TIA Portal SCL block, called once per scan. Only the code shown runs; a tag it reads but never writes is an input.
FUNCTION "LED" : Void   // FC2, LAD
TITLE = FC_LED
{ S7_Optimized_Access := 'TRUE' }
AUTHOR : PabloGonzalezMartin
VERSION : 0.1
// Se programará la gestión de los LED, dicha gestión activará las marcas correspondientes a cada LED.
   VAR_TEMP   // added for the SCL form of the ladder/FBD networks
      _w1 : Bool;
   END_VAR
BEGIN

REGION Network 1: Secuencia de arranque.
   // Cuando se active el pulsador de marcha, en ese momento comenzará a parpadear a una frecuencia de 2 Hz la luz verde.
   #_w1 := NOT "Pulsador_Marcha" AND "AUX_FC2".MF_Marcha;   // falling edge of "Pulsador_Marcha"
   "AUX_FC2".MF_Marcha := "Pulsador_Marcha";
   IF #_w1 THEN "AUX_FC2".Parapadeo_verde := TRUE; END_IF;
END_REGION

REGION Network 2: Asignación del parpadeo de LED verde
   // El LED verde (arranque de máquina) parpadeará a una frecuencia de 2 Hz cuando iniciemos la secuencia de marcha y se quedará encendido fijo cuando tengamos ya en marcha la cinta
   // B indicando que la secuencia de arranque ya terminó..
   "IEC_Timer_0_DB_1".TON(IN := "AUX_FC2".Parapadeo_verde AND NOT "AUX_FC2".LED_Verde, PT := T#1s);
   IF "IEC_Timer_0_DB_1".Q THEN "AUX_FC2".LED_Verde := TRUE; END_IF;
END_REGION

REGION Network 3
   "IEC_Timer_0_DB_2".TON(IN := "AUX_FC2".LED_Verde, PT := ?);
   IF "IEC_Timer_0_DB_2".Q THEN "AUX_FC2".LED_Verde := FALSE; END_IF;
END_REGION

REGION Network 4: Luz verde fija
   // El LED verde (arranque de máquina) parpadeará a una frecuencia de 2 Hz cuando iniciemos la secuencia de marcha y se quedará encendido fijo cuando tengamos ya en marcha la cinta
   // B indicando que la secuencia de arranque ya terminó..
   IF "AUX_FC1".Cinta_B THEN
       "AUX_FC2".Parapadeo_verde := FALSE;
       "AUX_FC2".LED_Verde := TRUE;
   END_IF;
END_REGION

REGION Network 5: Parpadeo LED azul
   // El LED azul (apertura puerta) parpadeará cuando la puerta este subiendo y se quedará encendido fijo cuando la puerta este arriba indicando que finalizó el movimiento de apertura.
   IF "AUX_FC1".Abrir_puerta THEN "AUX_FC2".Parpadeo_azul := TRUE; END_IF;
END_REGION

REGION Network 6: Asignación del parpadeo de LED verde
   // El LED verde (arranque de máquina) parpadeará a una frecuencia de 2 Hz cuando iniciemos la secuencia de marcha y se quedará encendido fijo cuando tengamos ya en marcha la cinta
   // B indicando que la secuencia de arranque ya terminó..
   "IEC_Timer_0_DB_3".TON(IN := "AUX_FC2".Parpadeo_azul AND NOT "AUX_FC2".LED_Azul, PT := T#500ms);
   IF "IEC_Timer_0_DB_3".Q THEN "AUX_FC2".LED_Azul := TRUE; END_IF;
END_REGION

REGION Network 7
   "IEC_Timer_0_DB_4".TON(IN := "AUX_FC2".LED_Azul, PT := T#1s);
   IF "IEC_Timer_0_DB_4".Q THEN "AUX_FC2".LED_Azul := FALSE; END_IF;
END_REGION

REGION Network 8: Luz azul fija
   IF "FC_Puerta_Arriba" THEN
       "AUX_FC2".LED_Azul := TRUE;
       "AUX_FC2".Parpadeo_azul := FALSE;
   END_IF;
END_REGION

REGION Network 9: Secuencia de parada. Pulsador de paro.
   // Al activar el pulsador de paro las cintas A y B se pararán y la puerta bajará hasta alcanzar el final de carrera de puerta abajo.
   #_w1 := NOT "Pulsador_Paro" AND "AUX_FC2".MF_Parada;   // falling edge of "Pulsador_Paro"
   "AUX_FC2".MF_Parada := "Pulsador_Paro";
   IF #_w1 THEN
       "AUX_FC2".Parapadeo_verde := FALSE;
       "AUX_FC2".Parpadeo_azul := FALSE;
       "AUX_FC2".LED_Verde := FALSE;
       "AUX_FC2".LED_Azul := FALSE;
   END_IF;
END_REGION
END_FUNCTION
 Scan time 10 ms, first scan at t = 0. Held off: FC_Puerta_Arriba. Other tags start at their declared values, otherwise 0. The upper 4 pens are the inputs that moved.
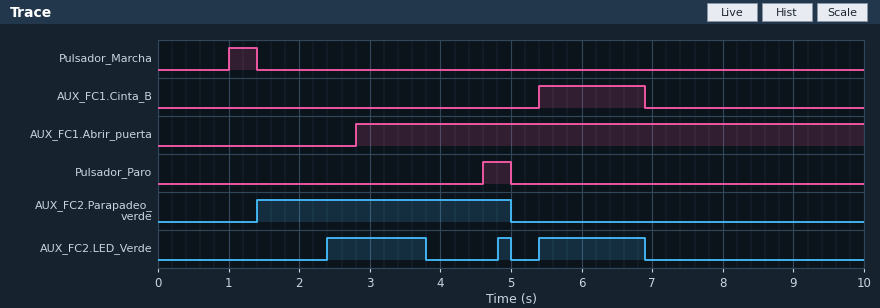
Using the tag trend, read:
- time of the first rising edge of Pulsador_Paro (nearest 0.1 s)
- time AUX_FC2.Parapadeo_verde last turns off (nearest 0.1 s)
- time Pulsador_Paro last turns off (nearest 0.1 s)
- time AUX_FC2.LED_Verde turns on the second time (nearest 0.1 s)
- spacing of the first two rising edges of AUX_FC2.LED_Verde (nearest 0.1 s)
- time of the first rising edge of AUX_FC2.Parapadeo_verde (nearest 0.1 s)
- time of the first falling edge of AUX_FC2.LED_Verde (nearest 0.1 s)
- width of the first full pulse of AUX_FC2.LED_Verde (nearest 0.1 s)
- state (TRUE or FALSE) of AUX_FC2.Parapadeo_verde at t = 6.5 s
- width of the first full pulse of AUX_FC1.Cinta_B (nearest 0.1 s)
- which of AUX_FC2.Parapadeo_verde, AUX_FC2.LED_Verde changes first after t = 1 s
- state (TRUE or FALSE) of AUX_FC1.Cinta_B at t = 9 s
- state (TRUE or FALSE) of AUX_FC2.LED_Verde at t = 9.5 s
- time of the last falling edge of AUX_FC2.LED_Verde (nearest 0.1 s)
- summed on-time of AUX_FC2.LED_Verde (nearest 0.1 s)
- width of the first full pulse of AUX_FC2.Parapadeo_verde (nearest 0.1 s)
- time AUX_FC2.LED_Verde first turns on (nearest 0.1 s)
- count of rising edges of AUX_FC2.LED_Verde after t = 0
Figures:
4.6 s
5.0 s
5.0 s
4.8 s
2.4 s
1.4 s
3.8 s
1.4 s
FALSE
1.5 s
AUX_FC2.Parapadeo_verde
FALSE
FALSE
6.9 s
3.1 s
3.6 s
2.4 s
3
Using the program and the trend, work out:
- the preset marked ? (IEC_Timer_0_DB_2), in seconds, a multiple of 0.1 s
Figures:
1.4 s
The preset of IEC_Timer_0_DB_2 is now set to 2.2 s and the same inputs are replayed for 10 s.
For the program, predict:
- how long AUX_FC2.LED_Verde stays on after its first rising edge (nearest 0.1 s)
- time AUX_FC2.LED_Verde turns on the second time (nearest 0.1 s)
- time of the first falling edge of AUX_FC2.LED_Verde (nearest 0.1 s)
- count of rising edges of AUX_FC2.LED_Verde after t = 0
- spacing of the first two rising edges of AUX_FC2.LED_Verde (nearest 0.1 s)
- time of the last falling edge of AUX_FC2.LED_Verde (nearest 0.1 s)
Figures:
2.2 s
5.4 s
4.6 s
2
3.0 s
7.6 s
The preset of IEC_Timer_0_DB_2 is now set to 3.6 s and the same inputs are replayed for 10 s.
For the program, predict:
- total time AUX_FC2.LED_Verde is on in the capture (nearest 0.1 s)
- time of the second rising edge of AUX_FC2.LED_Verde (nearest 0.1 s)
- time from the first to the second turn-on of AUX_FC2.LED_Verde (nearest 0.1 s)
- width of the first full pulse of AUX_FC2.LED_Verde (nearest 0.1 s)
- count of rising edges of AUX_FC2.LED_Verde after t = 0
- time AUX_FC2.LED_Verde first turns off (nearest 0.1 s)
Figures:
6.2 s
5.4 s
3.0 s
2.6 s
2
5.0 s
